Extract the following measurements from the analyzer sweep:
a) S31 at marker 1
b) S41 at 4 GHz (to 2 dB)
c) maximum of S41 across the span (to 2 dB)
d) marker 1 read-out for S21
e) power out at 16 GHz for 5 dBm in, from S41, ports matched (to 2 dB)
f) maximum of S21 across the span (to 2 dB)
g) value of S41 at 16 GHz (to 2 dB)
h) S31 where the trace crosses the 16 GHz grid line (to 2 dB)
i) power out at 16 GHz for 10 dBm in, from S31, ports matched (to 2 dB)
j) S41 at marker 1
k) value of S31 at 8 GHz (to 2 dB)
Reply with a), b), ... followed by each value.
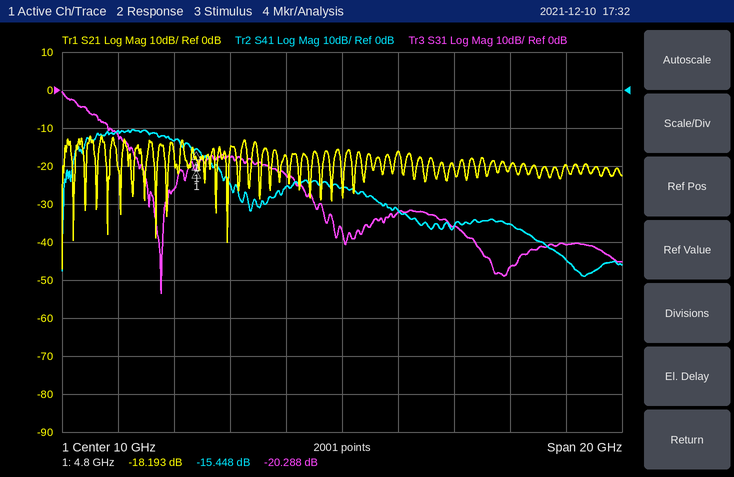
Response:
a) -20.288 dB
b) -14 dB
c) -10 dB
d) -18.193 dB
e) -30 dBm
f) -12 dB
g) -36 dB
h) -46 dB
i) -36 dBm
j) -15.448 dB
k) -22 dB
